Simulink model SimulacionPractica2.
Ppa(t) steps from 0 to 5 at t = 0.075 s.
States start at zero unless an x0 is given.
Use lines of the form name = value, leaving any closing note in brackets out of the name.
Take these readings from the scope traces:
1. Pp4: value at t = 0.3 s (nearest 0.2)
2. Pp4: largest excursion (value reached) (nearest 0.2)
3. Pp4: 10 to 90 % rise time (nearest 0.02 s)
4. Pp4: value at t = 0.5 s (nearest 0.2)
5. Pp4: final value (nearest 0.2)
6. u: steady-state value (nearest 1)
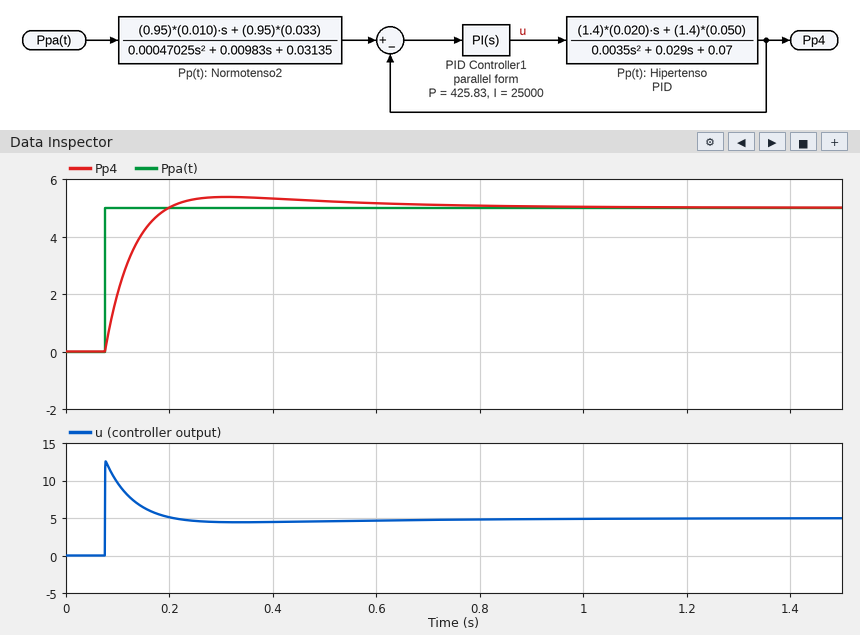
Pp4: value at t = 0.3 s = 5.4
Pp4: largest excursion (value reached) = 5.4
Pp4: 10 to 90 % rise time = 0.08 s
Pp4: value at t = 0.5 s = 5.2
Pp4: final value = 5.0
u: steady-state value = 5
